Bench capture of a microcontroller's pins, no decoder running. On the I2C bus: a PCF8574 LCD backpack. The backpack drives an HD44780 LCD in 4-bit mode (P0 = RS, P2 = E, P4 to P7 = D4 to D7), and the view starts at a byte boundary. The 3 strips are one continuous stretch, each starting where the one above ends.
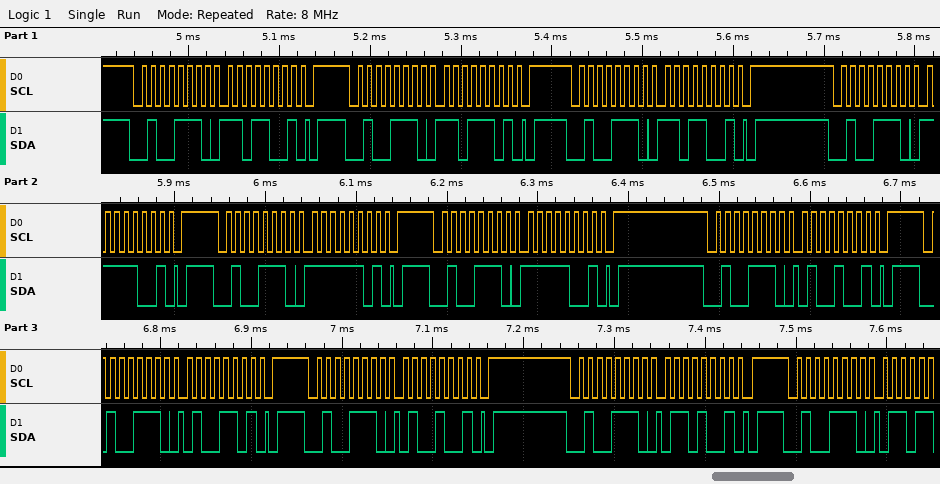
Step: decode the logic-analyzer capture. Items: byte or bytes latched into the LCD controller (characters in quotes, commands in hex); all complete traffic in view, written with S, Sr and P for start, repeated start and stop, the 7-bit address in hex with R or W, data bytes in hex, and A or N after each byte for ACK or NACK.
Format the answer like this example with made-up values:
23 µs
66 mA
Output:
data 0xDF
S 27W A D9 A P S 27W A DD A P S 27W A D9 A P S 27W A F9 A P S 27W A FD A P S 27W A F9 A P S 27W A 49 A P S 27W A 4D A P S 27W A 49 A P S 27W A 69 A P S 27W A
